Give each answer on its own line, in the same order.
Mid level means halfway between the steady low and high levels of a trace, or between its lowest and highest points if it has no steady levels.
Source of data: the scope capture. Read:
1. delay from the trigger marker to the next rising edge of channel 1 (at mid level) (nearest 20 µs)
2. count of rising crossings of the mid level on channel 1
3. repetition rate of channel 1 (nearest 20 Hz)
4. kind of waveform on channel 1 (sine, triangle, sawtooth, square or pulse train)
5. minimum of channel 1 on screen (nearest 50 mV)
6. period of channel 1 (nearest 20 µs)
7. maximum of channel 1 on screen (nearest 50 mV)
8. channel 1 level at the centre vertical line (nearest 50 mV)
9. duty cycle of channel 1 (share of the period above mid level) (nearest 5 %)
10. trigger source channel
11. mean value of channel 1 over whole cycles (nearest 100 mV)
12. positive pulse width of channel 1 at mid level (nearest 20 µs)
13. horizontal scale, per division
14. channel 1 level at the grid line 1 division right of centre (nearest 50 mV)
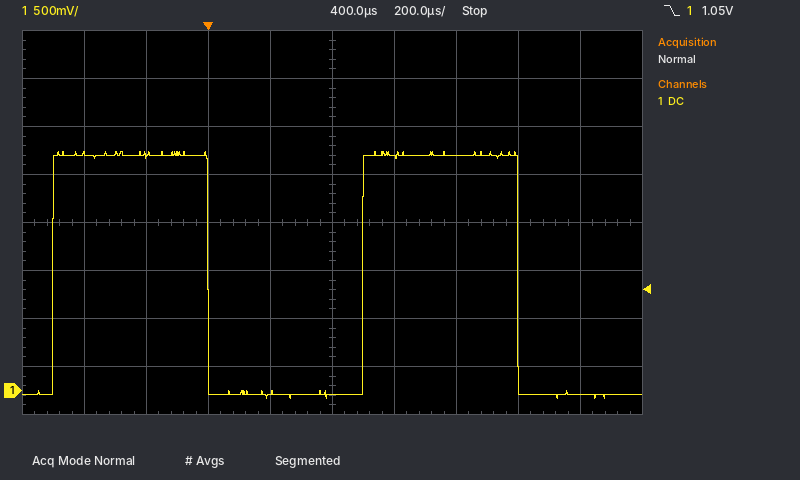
500 µs
2
1.00 kHz
square
-100 mV
1.00 ms
2.50 V
-50 mV
50 %
channel 1
1.2 V
500 µs
200 µs
2.45 V
